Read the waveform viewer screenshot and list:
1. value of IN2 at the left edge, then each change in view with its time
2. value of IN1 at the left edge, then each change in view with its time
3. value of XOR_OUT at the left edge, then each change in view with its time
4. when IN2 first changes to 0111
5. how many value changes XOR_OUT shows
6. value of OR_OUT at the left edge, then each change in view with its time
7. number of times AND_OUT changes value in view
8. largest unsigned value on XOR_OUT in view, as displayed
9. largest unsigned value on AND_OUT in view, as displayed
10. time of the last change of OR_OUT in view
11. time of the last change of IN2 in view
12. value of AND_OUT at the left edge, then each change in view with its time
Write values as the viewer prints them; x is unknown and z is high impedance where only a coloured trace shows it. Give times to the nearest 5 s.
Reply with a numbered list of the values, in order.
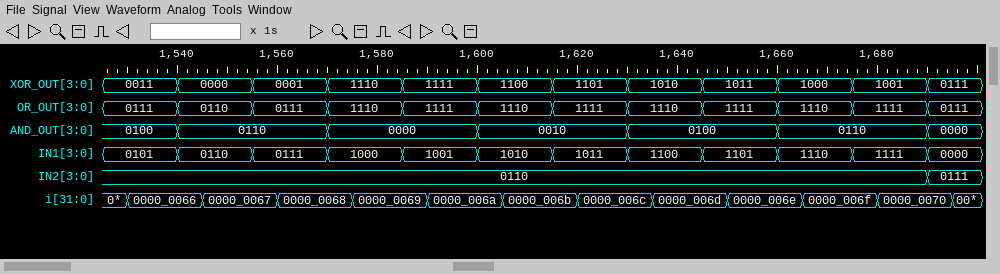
1. 0110, 0111 at 1690 s
2. 0101, 0110 at 1540 s, 0111 at 1555 s, 1000 at 1570 s, 1001 at 1585 s, 1010 at 1600 s, 1011 at 1615 s, 1100 at 1630 s, 1101 at 1645 s, 1110 at 1660 s, 1111 at 1675 s, 0000 at 1690 s
3. 0011, 0000 at 1540 s, 0001 at 1555 s, 1110 at 1570 s, 1111 at 1585 s, 1100 at 1600 s, 1101 at 1615 s, 1010 at 1630 s, 1011 at 1645 s, 1000 at 1660 s, 1001 at 1675 s, 0111 at 1690 s
4. 1690 s
5. 11
6. 0111, 0110 at 1540 s, 0111 at 1555 s, 1110 at 1570 s, 1111 at 1585 s, 1110 at 1600 s, 1111 at 1615 s, 1110 at 1630 s, 1111 at 1645 s, 1110 at 1660 s, 1111 at 1675 s, 0111 at 1690 s
7. 6
8. 1111
9. 0110
10. 1690 s
11. 1690 s
12. 0100, 0110 at 1540 s, 0000 at 1570 s, 0010 at 1600 s, 0100 at 1630 s, 0110 at 1660 s, 0000 at 1690 s
